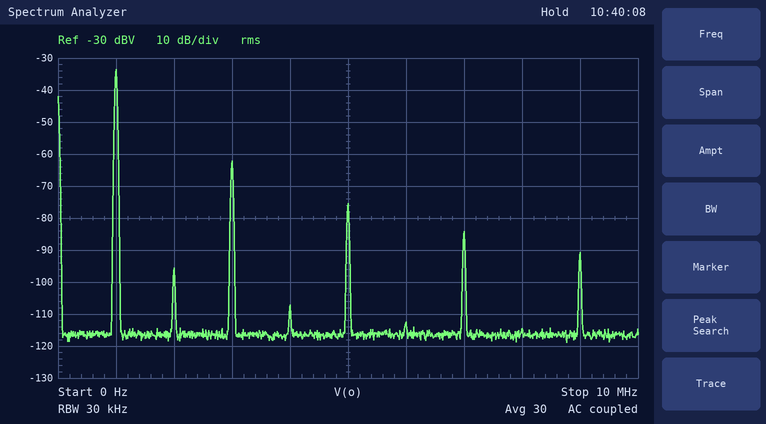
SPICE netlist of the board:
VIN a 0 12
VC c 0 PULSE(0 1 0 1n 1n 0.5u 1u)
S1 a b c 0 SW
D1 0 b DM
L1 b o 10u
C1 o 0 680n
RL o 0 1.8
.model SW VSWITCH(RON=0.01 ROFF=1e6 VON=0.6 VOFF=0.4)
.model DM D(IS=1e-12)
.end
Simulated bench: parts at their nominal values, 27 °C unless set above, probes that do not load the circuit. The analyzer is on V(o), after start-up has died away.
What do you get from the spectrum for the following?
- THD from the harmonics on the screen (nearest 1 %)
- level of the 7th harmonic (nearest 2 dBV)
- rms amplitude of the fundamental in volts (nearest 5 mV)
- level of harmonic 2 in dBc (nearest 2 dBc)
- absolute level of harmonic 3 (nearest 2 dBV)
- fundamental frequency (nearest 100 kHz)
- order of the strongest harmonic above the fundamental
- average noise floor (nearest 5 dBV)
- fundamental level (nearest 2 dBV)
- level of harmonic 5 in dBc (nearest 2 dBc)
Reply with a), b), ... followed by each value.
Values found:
a) 4 %
b) -84 dBV
c) 20 mV
d) -62 dBc
e) -62 dBV
f) 1.0 MHz
g) 3
h) -115 dBV
i) -34 dBV
j) -42 dBc
